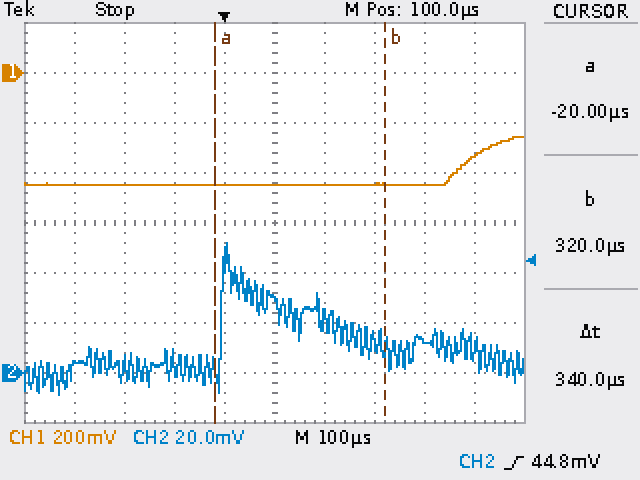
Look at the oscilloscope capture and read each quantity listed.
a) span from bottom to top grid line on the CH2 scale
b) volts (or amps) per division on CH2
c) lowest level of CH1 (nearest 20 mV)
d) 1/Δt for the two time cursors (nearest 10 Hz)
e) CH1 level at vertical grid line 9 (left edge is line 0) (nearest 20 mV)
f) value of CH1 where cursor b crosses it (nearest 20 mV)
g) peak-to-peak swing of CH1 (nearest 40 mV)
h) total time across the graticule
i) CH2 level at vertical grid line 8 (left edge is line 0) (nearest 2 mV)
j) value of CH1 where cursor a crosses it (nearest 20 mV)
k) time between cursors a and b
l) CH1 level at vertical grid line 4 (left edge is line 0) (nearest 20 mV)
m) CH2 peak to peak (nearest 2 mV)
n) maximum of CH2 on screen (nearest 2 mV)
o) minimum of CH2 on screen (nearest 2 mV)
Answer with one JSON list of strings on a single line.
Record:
["160 mV", "20 mV", "-440 mV", "2.94 kHz", "-340 mV", "-440 mV", "200 mV", "1 ms", "14 mV", "-440 mV", "340 µs", "-440 mV", "60 mV", "52 mV", "-8 mV"]
